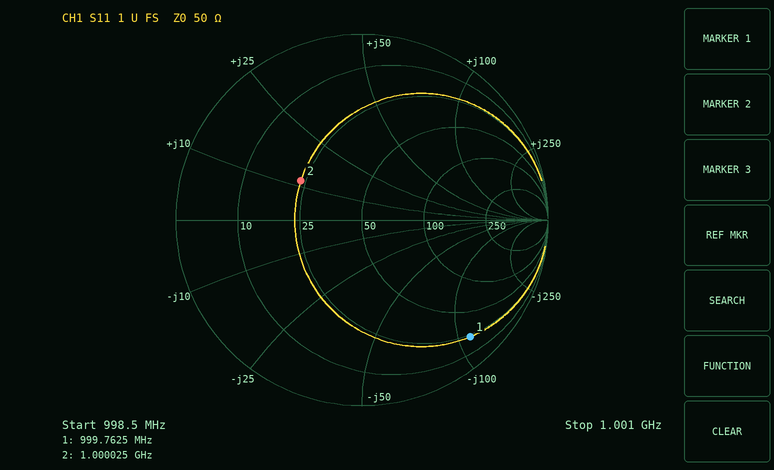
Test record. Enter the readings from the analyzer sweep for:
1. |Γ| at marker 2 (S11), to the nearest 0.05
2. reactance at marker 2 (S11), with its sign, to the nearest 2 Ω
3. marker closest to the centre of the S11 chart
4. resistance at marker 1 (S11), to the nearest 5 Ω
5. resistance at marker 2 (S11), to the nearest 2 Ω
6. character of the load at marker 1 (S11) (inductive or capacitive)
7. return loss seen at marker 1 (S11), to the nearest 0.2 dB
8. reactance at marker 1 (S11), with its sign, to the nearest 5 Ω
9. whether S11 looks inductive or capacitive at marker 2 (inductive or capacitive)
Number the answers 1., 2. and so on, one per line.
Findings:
1. 0.40
2. +12 Ω
3. marker 2
4. 25 Ω
5. 24 Ω
6. capacitive
7. 1.4 dB
8. -110 Ω
9. inductive
